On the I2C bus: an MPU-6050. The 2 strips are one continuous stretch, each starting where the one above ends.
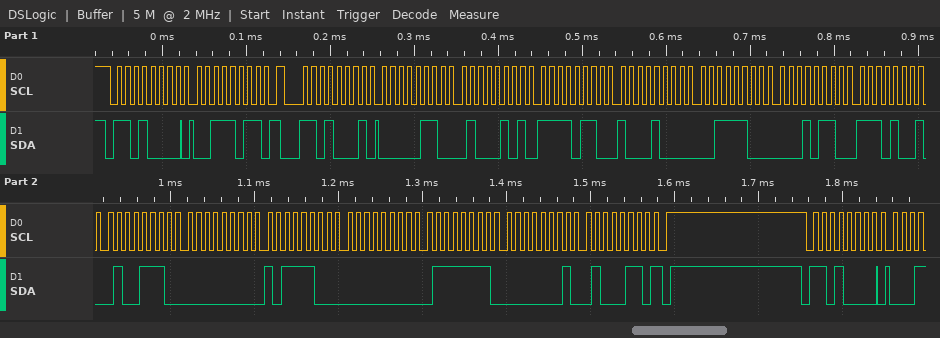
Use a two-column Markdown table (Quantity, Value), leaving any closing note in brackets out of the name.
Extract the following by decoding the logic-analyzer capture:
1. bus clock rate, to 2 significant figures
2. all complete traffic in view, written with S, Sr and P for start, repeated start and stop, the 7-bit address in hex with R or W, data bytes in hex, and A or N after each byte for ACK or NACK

| Quantity | Value |
|---|---|
| bus clock rate, to 2 significant figures | 100 kHz |
| all complete traffic in view, written with S, Sr and P for start, repeated start and stop, the 7-bit address in hex with R or W, data bytes in hex, and A or N after each byte for ACK or NACK | S 68W A 3B A Sr 68R A 06 A 45 A F6 A 88 A 3C A 16 A E9 A 4E A 00 A BC A 00 A 7F A 01 A 46 N P S 68W A |
